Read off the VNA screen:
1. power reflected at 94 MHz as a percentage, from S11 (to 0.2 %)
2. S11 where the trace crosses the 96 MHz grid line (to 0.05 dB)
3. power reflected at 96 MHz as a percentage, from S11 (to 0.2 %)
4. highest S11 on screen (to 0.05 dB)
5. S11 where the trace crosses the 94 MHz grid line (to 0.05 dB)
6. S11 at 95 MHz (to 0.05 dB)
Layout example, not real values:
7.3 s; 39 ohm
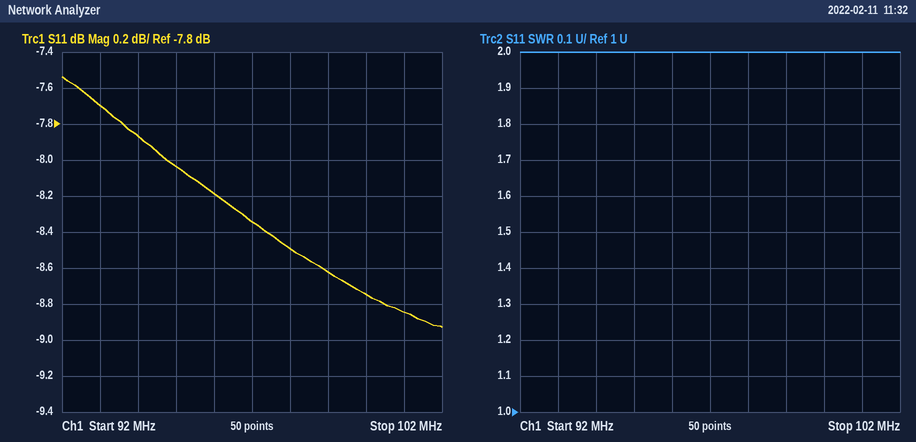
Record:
16.4 %; -8.20 dB; 15.2 %; -7.55 dB; -7.85 dB; -8.05 dB
